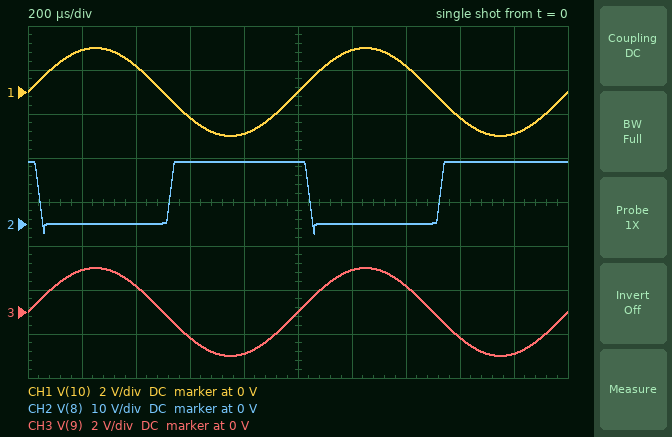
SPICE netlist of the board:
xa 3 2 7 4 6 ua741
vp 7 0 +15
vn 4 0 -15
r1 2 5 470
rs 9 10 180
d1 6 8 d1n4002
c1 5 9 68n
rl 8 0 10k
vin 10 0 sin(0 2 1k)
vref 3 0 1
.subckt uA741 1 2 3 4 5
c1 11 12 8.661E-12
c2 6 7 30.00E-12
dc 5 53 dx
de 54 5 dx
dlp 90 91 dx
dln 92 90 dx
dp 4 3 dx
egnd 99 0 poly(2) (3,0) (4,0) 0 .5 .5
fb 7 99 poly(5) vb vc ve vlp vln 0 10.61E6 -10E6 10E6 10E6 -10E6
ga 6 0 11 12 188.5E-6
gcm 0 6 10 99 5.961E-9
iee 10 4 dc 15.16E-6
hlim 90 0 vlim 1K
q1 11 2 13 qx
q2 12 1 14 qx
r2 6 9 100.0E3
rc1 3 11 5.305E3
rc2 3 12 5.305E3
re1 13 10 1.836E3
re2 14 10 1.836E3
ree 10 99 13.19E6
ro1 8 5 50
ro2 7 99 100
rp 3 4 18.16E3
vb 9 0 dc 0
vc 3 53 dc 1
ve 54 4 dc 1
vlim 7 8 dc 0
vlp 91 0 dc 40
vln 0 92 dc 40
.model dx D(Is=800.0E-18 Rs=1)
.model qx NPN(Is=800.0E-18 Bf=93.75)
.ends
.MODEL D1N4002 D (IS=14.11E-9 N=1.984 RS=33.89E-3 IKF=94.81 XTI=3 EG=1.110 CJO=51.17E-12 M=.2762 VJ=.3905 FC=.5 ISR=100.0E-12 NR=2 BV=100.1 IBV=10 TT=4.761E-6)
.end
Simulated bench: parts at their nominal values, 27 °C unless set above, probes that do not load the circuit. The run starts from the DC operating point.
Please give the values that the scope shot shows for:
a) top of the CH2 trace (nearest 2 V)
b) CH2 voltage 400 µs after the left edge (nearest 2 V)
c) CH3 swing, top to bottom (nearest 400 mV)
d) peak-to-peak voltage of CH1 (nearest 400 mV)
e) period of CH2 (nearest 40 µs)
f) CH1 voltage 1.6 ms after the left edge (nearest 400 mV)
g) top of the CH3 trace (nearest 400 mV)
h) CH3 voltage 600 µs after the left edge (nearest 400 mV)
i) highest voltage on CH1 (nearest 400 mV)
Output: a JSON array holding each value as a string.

["14 V", "0 V", "4.0 V", "4.0 V", "1.00 ms", "-1.2 V", "2.0 V", "-1.2 V", "2.0 V"]
